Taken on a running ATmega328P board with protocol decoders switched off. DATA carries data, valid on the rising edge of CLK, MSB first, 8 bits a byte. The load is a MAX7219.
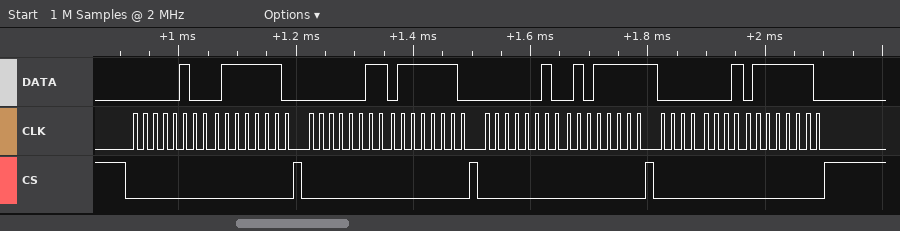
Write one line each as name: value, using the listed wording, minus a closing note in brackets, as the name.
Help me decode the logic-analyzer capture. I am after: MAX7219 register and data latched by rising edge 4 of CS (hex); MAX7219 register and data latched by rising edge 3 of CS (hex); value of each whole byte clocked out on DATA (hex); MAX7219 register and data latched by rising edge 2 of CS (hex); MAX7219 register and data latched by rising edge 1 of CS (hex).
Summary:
MAX7219 register and data latched by rising edge 4 of CS: register 0x1, data 0x7E
MAX7219 register and data latched by rising edge 3 of CS: register 0x2, data 0x5F
value of each whole byte clocked out on DATA: 04 7E 03 7E 02 5F 01 7E
MAX7219 register and data latched by rising edge 2 of CS: register 0x3, data 0x7E
MAX7219 register and data latched by rising edge 1 of CS: register 0x4, data 0x7E
